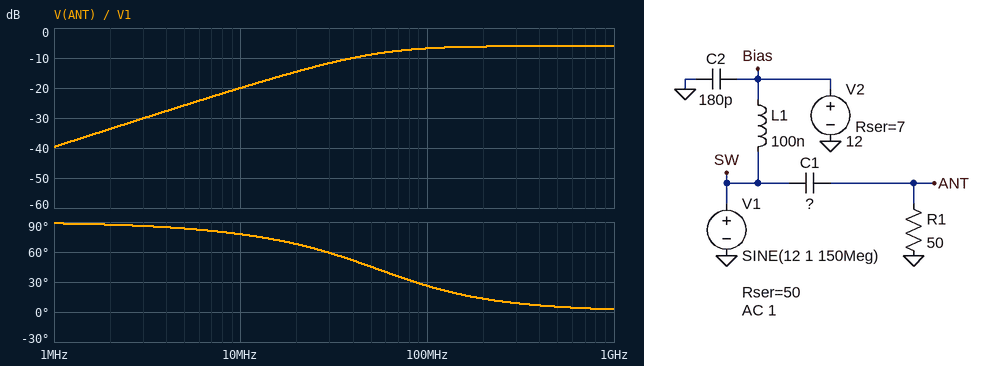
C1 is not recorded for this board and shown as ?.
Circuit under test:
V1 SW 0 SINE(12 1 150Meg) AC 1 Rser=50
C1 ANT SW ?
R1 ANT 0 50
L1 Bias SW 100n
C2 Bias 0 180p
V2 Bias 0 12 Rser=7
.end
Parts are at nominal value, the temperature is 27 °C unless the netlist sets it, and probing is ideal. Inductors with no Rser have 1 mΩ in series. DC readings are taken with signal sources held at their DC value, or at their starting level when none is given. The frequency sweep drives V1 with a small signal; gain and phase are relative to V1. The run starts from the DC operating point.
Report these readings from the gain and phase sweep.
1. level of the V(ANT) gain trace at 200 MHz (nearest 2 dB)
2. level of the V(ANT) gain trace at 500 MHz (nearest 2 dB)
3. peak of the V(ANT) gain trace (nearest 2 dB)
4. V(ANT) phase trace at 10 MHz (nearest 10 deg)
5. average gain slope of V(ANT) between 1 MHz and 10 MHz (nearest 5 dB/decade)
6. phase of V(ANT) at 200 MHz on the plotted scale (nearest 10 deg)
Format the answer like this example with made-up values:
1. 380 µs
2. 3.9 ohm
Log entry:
1. -6 dB
2. -6 dB
3. -6 dB
4. 80 deg
5. 20 dB/decade
6. 10 deg
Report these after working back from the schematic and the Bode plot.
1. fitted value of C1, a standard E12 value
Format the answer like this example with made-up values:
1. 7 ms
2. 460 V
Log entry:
1. 270 pF
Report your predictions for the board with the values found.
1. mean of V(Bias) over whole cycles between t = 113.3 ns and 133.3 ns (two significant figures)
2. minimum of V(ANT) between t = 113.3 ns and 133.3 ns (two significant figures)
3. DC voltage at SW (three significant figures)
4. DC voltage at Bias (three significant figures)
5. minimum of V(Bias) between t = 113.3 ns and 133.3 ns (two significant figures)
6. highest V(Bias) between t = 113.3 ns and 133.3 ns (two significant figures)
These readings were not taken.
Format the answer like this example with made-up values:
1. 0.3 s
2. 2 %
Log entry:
1. 12 V
2. -480 mV
3. 12.0 V
4. 12.0 V
5. 12 V
6. 12 V
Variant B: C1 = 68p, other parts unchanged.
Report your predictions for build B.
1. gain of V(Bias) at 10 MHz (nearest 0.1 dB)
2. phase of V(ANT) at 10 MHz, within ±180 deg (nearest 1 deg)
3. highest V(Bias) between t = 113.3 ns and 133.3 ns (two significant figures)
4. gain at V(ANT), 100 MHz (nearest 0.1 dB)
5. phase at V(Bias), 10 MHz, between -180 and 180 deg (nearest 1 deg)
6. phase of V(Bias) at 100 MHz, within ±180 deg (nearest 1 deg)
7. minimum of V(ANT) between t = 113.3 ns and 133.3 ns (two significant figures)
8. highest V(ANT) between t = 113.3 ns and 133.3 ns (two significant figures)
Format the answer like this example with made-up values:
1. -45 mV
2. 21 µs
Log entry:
1. -18.2 dB
2. 110 deg
3. 12 V
4. -6.6 dB
5. -12 deg
6. -111 deg
7. -490 mV
8. 490 mV
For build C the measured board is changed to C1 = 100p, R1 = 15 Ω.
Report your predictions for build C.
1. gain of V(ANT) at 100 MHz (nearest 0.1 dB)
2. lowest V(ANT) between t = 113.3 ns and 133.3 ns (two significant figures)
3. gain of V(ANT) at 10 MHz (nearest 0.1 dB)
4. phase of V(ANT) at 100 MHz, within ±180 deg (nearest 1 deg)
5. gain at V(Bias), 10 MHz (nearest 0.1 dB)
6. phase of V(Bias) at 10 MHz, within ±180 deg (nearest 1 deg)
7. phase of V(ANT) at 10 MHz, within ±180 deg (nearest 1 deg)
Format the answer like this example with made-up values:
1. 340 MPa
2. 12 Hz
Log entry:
1. -12.1 dB
2. -240 mV
3. -36.4 dB
4. 29 deg
5. -18.1 dB
6. -13 deg
7. 116 deg
